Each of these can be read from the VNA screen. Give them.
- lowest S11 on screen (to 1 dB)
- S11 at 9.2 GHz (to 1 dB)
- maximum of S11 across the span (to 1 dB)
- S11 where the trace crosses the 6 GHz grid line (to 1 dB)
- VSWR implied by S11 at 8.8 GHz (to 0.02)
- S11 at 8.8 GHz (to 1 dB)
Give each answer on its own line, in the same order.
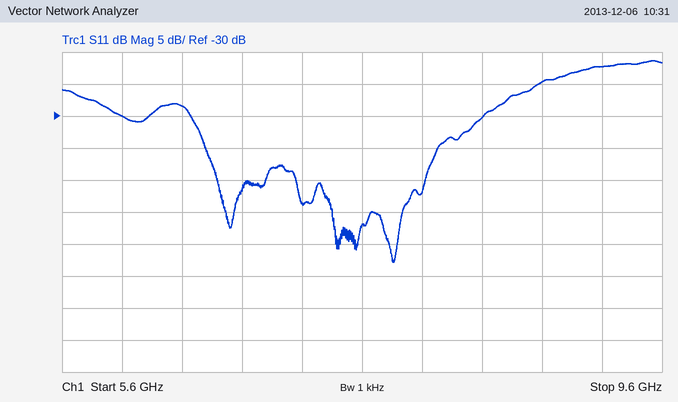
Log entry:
-53 dB
-22 dB
-21 dB
-30 dB
1.12
-25 dB
